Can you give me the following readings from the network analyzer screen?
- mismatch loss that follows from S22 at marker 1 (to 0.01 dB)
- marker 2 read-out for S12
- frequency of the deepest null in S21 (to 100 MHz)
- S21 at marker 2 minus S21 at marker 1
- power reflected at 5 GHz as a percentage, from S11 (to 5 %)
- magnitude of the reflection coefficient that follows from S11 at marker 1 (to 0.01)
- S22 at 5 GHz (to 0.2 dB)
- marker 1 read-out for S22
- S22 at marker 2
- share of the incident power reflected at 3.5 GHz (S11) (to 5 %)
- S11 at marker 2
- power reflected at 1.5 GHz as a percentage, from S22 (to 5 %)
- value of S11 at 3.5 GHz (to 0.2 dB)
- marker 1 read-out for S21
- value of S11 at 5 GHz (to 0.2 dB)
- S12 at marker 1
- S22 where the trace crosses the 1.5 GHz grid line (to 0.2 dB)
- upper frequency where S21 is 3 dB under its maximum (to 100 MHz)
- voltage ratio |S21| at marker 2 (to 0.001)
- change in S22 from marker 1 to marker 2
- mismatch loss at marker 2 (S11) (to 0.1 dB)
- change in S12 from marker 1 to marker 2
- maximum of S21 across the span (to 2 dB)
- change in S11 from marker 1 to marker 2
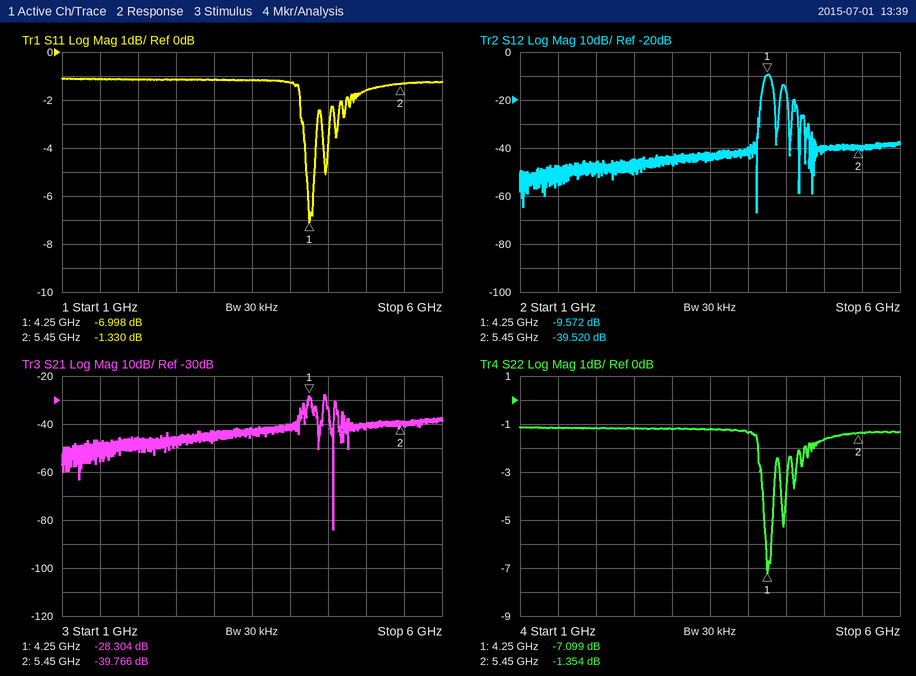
0.94 dB
-39.520 dB
4.6 GHz
-11.462 dB
70 %
0.45
-1.6 dB
-7.099 dB
-1.354 dB
75 %
-1.330 dB
75 %
-1.2 dB
-28.304 dB
-1.6 dB
-9.572 dB
-1.2 dB
4.5 GHz
0.010
5.745 dB
5.8 dB
-29.948 dB
-28 dB
5.668 dB
